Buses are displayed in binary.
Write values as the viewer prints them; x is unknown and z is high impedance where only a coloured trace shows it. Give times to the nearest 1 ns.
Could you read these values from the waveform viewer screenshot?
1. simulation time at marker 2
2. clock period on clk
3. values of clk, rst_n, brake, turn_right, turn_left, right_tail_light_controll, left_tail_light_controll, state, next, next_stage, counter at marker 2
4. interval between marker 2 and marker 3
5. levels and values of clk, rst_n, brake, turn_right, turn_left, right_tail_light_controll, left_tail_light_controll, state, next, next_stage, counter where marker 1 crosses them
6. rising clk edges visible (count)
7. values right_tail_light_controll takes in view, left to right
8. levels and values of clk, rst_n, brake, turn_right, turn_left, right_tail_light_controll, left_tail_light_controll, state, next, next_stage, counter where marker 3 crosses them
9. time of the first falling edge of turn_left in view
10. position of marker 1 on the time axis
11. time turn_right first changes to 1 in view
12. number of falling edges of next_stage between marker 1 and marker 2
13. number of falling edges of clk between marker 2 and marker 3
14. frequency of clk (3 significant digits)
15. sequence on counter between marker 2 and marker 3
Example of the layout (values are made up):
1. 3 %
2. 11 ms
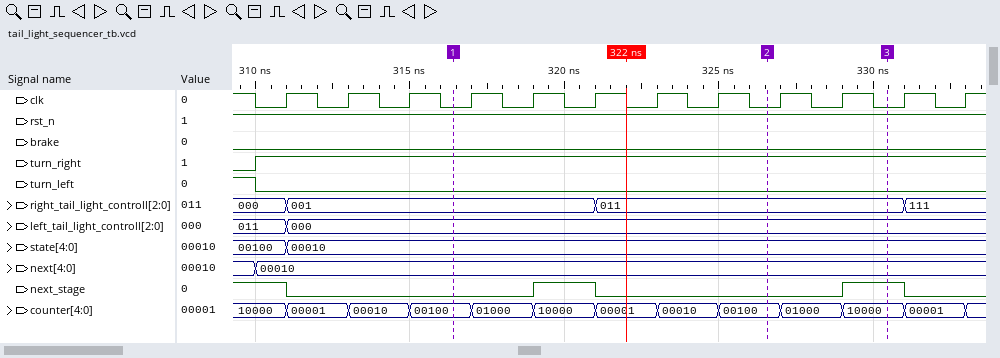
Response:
1. 327 ns
2. 2 ns
3. clk=0, rst_n=1, brake=0, turn_right=1, turn_left=0, right_tail_light_controll=011, left_tail_light_controll=000, state=00010, next=00010, next_stage=0, counter=00100
4. 4 ns
5. clk=0, rst_n=1, brake=0, turn_right=1, turn_left=0, right_tail_light_controll=001, left_tail_light_controll=000, state=00010, next=00010, next_stage=0, counter=00100
6. 12
7. 000, 001, 011, 111
8. clk=0, rst_n=1, brake=0, turn_right=1, turn_left=0, right_tail_light_controll=011, left_tail_light_controll=000, state=00010, next=00010, next_stage=1, counter=10000
9. 310 ns
10. 316 ns
11. 310 ns
12. 1
13. 2
14. 500 MHz
15. 00100, 01000, 10000
